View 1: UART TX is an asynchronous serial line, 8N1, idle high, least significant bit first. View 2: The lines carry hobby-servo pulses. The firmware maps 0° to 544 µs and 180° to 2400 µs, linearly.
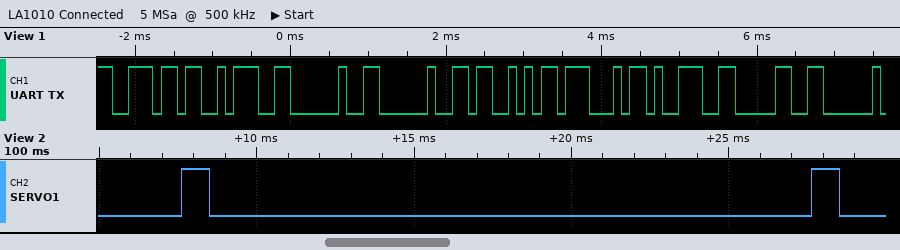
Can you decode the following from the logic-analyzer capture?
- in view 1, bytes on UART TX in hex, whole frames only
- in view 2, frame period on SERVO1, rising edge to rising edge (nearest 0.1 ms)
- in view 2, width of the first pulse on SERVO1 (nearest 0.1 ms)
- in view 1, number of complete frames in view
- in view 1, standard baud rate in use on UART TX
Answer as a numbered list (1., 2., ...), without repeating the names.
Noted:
1. 6E 3A 20 20 53 47 39 30
2. 20.0 ms
3. 0.9 ms
4. 8
5. 9600 baud
